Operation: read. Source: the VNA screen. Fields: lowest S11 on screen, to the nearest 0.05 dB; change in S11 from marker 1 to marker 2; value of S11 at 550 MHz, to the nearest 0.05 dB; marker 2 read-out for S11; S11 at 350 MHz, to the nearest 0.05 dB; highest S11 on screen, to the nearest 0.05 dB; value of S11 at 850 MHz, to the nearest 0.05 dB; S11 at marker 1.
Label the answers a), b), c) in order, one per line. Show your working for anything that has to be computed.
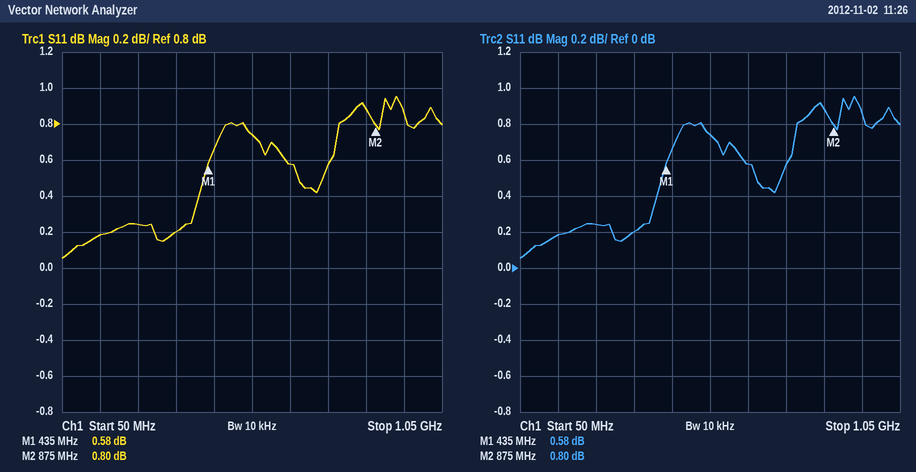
a) 0.05 dB
b) 0.8 − (0.58) = 0.22 dB
c) 0.75 dB
d) 0.80 dB
e) 0.20 dB
f) 0.95 dB
g) 0.90 dB
h) 0.58 dB
